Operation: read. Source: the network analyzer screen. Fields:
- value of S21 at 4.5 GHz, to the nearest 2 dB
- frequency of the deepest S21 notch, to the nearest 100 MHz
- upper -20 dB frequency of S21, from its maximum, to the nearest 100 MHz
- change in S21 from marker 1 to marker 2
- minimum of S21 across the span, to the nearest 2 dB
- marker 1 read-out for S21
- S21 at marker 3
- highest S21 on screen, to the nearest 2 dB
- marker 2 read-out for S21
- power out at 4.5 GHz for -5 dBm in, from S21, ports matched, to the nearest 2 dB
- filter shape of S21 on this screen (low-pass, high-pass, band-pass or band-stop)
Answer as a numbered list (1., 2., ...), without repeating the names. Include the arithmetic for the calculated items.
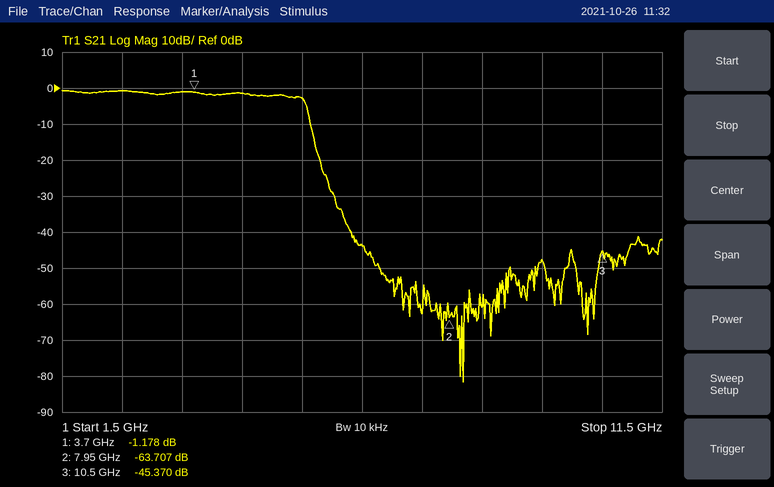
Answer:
1. -2 dB
2. 8.2 GHz
3. 5.8 GHz
4. -63.707 − (-1.178) = -62.529 dB
5. -82 dB
6. -1.178 dB
7. -45.370 dB
8. 0 dB
9. -63.707 dB
10. -5 dBm + (-2 dB) = -6 dBm
11. low-pass
